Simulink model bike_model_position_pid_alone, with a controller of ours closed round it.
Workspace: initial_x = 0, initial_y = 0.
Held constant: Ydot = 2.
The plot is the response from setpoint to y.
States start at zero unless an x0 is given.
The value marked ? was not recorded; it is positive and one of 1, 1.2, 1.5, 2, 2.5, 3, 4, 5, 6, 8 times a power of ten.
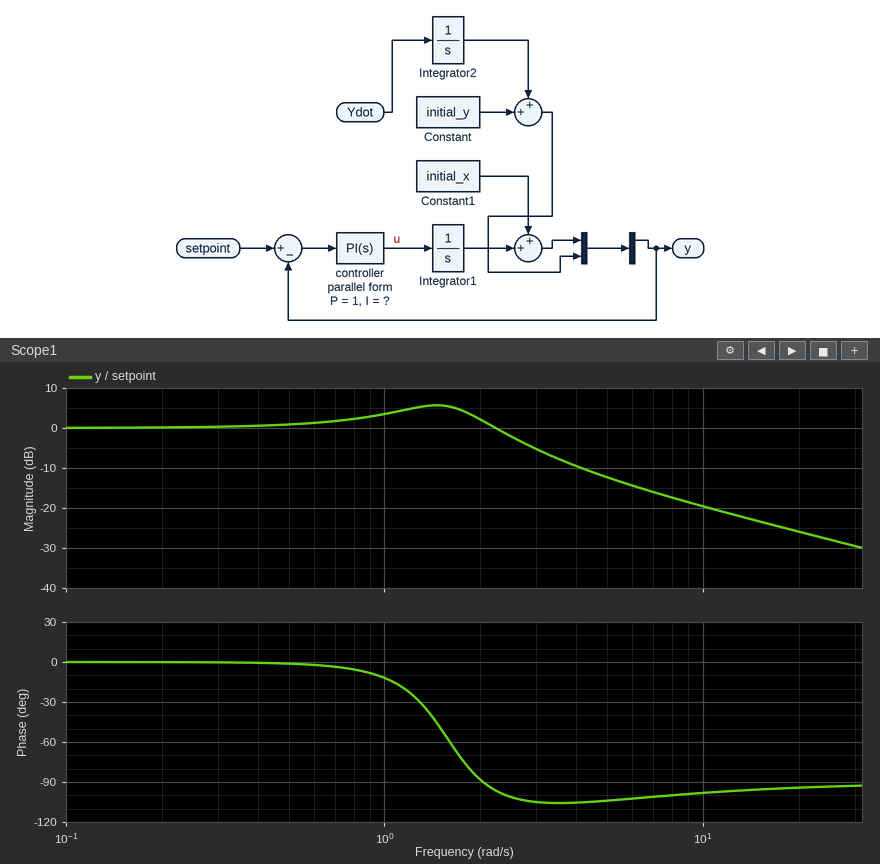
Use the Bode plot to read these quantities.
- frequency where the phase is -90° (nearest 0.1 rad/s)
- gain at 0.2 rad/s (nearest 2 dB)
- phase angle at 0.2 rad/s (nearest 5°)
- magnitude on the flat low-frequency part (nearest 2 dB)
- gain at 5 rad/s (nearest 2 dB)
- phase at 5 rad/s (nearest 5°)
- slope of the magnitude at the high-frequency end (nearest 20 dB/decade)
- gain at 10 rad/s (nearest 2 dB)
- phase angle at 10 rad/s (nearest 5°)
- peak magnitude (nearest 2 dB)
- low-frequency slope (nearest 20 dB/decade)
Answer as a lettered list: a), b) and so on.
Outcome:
a) 2.0 rad/s
b) 0 dB
c) 0°
d) 0 dB
e) -12 dB
f) -105°
g) -20 dB/decade
h) -20 dB
i) -100°
j) 6 dB
k) 0 dB/decade
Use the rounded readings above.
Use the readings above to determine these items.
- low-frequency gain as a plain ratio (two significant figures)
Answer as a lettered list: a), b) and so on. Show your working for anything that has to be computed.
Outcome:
a) 10^(0 / 20) = 1.0
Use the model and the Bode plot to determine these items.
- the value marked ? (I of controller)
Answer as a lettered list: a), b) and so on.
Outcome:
a) 2.5
